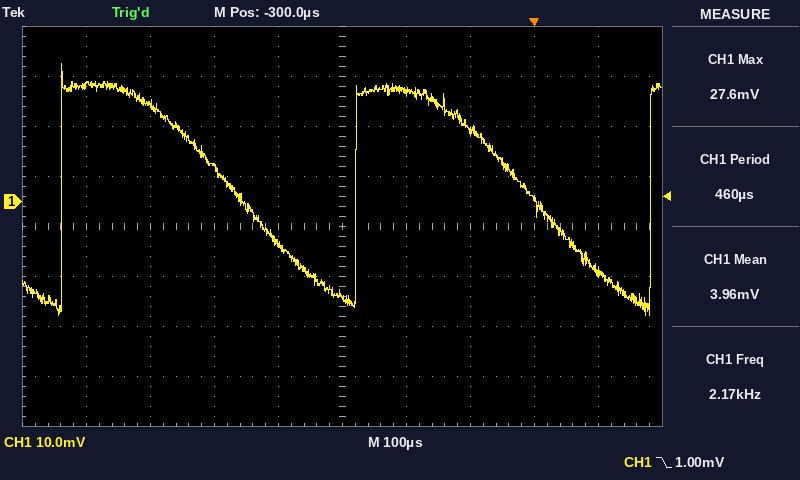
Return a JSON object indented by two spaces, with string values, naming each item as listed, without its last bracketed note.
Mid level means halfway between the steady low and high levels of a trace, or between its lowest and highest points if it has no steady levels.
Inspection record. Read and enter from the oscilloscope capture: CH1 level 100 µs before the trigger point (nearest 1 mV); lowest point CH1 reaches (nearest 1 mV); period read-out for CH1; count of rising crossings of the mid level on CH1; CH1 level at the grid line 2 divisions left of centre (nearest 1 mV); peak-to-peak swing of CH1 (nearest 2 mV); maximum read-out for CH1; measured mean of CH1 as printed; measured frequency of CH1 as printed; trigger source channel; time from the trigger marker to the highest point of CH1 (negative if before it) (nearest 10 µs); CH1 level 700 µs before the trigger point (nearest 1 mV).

{
  "CH1 level 100 µs before the trigger point": "14 mV",
  "lowest point CH1 reaches": "-23 mV",
  "period read-out for CH1": "460 µs",
  "count of rising crossings of the mid level on CH1": "3",
  "CH1 level at the grid line 2 divisions left of centre": "7 mV",
  "peak-to-peak swing of CH1": "50 mV",
  "maximum read-out for CH1": "27.6 mV",
  "measured mean of CH1 as printed": "3.96 mV",
  "measured frequency of CH1 as printed": "2.17 kHz",
  "trigger source channel": "CH1",
  "time from the trigger marker to the highest point of CH1 (negative if before it)": "-740 µs",
  "CH1 level 700 µs before the trigger point": "23 mV"
}
